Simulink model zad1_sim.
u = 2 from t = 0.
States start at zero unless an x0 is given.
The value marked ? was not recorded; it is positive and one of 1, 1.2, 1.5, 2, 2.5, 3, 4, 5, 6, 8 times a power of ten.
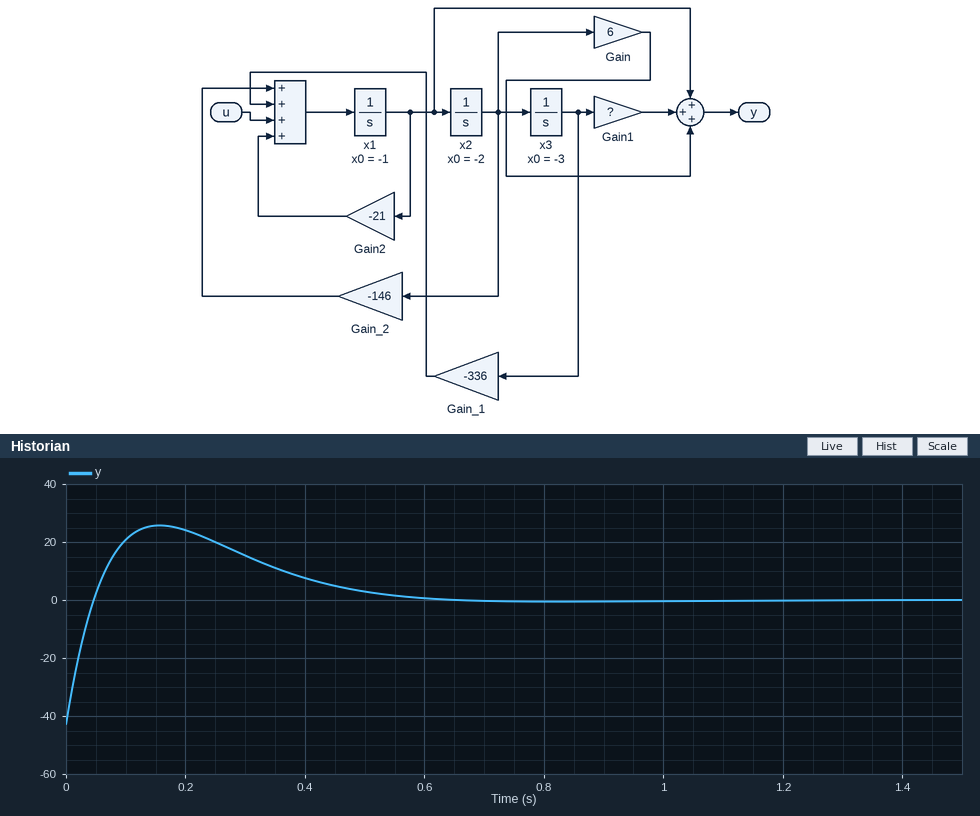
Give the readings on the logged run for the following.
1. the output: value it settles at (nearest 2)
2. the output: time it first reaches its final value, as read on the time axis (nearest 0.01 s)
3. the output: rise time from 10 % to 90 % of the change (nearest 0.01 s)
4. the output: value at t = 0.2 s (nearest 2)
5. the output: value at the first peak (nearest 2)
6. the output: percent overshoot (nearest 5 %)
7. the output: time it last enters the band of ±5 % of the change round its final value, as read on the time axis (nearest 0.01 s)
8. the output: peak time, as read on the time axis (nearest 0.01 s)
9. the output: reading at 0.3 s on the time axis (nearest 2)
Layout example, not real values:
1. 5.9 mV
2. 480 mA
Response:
1. 0
2. 0.05 s
3. 0.04 s
4. 24
5. 26
6. 60 %
7. 0.52 s
8. 0.16 s
9. 16
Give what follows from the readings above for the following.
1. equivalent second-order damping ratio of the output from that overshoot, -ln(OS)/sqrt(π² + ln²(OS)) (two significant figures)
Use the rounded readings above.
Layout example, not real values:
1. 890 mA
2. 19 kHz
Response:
1. 0.16
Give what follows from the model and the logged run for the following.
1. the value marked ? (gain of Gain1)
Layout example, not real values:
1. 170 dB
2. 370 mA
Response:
1. 10
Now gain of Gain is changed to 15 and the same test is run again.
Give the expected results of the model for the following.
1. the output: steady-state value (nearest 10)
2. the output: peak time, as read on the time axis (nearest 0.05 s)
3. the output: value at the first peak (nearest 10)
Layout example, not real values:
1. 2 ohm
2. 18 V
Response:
1. 0
2. 0.25 s
3. 70
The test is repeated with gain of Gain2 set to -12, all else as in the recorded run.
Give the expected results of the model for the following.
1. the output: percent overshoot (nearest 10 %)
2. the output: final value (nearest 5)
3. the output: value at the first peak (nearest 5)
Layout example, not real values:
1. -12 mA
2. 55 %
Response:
1. 120 %
2. 0
3. 50
